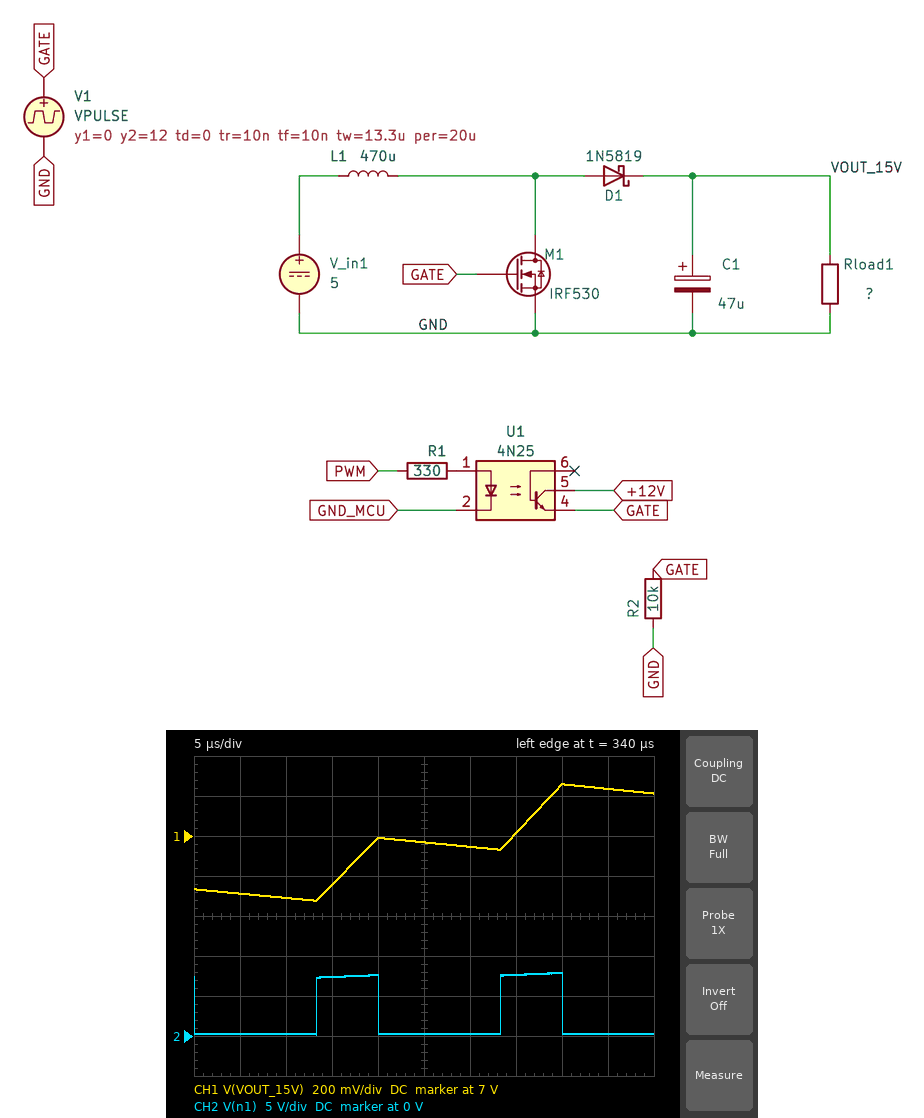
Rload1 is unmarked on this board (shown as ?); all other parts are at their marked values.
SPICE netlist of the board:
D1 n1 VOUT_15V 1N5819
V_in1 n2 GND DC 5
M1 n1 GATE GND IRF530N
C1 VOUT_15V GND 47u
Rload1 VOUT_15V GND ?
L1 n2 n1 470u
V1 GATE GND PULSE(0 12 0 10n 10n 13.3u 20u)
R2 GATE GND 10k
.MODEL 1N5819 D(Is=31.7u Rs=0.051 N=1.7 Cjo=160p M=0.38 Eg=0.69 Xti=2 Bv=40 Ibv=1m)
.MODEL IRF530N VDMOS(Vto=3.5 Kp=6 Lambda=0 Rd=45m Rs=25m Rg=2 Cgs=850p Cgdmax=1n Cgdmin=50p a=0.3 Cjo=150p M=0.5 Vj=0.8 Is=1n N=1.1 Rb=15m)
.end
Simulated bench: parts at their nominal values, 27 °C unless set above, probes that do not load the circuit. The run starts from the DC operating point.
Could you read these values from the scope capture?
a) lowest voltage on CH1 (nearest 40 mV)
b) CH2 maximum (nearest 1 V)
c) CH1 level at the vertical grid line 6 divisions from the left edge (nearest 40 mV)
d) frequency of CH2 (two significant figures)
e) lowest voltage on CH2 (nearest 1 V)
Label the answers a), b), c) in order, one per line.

a) 6.68 V
b) 8 V
c) 6.96 V
d) 50 kHz
e) 0 V
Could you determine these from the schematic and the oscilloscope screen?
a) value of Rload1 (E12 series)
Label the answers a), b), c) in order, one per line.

a) 33 Ω
